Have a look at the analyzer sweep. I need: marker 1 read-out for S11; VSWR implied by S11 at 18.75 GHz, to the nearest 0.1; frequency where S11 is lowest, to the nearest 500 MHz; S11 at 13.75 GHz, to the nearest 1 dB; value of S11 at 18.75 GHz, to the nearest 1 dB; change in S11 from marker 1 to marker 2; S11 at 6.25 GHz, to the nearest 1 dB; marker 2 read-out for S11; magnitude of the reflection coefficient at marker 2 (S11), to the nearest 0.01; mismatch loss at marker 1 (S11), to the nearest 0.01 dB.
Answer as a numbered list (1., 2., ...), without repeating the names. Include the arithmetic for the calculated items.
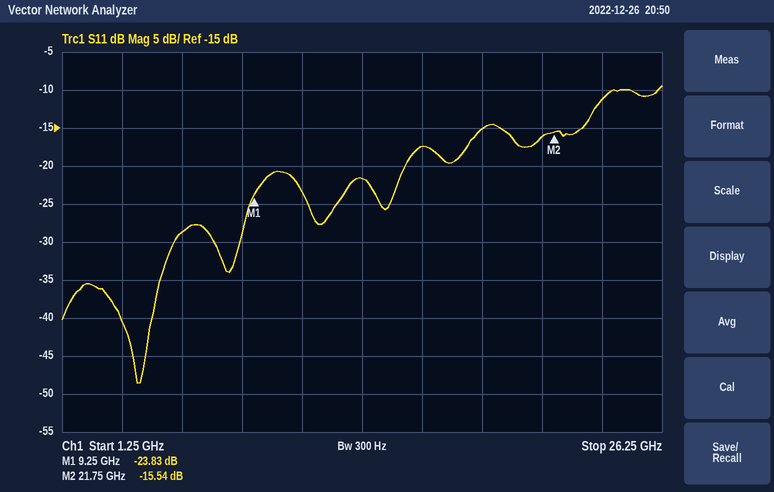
1. -23.83 dB
2. |Γ| = 10^(-15/20) = 0.1778; VSWR = (1 + 0.1778)/(1 − 0.1778) ≈ 1.4
3. 4.5 GHz
4. -22 dB
5. -15 dB
6. -15.54 − (-23.83) = 8.29 dB
7. -29 dB
8. -15.54 dB
9. 10^(-15.54/20) ≈ 0.17
10. −10 log10(1 − 10^(-23.83/10)) ≈ 0.02 dB
